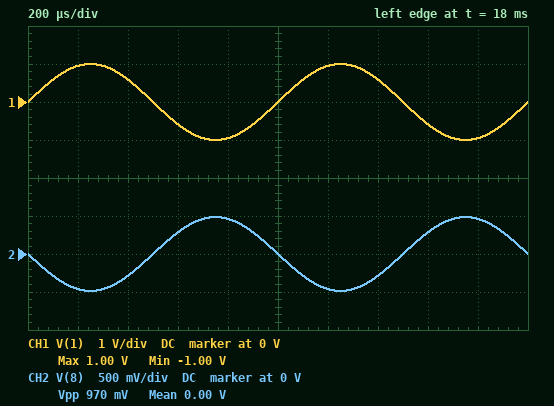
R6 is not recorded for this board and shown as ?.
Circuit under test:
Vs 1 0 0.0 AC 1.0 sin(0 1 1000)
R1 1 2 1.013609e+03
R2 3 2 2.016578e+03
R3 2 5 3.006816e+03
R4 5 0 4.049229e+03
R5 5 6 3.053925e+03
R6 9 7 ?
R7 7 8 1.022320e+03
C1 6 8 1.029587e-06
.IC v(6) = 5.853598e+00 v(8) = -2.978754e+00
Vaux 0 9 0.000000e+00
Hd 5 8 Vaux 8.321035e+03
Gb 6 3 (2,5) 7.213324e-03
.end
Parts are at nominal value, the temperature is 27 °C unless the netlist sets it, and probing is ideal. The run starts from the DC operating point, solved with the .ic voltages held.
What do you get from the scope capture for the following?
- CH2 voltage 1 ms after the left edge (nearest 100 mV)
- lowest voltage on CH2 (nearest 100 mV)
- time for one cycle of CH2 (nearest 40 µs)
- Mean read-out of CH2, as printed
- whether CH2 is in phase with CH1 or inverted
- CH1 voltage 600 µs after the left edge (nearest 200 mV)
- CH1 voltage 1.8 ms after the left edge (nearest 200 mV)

0 V
-500 mV
1.00 ms
0.00 V
inverted
-600 mV
-1.0 V
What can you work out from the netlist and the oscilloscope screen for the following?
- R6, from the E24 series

1.8 kΩ
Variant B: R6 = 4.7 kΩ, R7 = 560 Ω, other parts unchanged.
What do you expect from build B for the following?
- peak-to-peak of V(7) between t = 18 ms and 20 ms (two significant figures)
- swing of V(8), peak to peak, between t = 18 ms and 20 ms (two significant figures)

3.3 V
3.7 V
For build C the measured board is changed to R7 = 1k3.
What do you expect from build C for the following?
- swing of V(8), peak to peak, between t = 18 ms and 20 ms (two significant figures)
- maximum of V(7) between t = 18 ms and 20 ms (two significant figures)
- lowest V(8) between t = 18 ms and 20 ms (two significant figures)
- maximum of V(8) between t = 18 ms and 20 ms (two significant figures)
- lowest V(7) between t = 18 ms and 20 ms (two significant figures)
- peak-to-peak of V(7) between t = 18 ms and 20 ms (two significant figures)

1.1 V
330 mV
-570 mV
570 mV
-330 mV
660 mV
